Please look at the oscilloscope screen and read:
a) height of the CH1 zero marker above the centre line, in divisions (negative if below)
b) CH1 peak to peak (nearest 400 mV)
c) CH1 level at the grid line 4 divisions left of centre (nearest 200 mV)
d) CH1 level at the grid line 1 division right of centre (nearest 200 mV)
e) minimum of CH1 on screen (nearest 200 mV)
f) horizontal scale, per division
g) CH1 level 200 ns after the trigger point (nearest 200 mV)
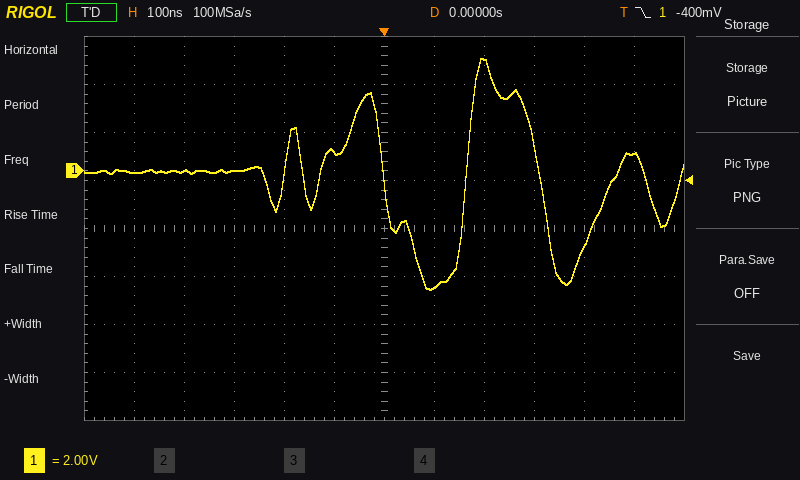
+1.2 div
9.6 V
0.0 V
-4.8 V
-5.0 V
100 ns
4.6 V
